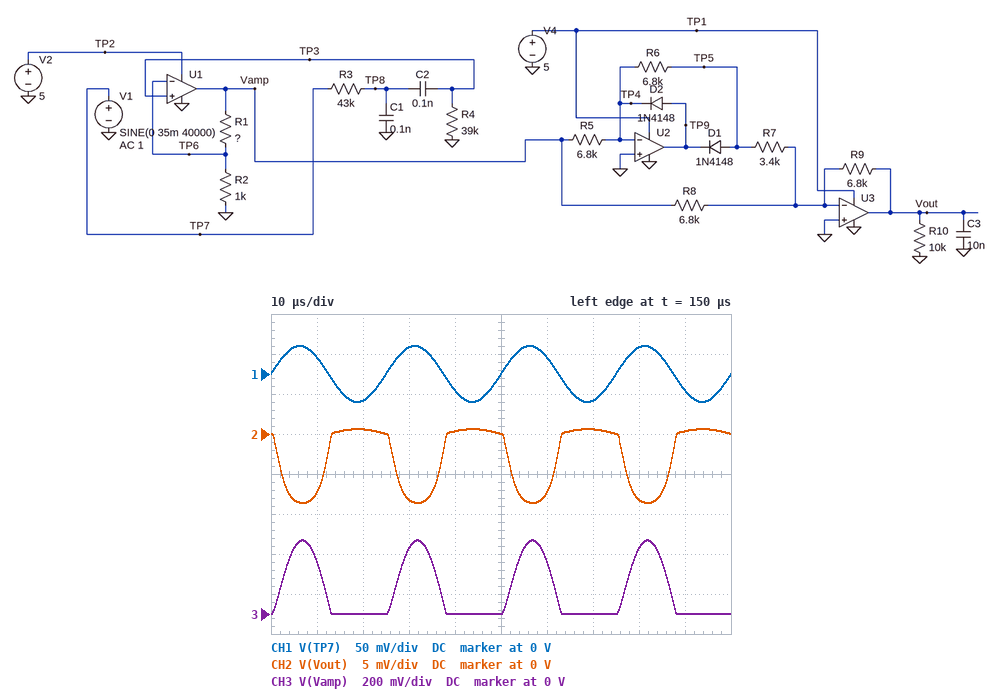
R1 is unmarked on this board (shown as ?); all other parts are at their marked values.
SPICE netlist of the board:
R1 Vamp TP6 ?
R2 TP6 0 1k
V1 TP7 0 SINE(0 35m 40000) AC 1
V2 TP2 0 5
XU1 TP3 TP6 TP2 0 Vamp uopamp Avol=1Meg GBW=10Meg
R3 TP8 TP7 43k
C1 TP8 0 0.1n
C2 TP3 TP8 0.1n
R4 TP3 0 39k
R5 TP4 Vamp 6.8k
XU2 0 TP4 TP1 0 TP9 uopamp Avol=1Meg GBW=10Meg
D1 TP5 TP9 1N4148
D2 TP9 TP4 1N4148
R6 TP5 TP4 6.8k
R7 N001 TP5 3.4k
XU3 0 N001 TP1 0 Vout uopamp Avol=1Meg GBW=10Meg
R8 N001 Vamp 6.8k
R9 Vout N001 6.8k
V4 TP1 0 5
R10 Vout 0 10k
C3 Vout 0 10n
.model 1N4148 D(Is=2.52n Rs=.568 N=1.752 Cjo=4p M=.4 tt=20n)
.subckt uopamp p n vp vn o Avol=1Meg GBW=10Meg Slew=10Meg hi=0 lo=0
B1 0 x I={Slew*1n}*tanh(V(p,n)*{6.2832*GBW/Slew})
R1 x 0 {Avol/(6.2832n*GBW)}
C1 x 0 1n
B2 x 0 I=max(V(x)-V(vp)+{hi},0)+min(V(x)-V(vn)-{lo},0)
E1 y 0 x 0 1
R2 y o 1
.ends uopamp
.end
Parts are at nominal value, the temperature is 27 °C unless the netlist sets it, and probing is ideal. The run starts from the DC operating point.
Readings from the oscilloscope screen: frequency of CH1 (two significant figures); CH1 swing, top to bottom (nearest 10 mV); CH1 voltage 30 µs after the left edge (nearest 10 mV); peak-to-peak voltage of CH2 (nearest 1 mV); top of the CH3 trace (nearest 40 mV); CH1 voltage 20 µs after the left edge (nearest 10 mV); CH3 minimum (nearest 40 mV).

40 kHz
70 mV
30 mV
9 mV
360 mV
-30 mV
0 V
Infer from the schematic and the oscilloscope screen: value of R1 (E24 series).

33 kΩ
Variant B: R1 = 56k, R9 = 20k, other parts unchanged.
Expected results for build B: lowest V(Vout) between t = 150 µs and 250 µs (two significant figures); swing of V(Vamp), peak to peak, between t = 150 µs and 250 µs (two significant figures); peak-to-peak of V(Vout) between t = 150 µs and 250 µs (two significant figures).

-9.9 mV
610 mV
12 mV
